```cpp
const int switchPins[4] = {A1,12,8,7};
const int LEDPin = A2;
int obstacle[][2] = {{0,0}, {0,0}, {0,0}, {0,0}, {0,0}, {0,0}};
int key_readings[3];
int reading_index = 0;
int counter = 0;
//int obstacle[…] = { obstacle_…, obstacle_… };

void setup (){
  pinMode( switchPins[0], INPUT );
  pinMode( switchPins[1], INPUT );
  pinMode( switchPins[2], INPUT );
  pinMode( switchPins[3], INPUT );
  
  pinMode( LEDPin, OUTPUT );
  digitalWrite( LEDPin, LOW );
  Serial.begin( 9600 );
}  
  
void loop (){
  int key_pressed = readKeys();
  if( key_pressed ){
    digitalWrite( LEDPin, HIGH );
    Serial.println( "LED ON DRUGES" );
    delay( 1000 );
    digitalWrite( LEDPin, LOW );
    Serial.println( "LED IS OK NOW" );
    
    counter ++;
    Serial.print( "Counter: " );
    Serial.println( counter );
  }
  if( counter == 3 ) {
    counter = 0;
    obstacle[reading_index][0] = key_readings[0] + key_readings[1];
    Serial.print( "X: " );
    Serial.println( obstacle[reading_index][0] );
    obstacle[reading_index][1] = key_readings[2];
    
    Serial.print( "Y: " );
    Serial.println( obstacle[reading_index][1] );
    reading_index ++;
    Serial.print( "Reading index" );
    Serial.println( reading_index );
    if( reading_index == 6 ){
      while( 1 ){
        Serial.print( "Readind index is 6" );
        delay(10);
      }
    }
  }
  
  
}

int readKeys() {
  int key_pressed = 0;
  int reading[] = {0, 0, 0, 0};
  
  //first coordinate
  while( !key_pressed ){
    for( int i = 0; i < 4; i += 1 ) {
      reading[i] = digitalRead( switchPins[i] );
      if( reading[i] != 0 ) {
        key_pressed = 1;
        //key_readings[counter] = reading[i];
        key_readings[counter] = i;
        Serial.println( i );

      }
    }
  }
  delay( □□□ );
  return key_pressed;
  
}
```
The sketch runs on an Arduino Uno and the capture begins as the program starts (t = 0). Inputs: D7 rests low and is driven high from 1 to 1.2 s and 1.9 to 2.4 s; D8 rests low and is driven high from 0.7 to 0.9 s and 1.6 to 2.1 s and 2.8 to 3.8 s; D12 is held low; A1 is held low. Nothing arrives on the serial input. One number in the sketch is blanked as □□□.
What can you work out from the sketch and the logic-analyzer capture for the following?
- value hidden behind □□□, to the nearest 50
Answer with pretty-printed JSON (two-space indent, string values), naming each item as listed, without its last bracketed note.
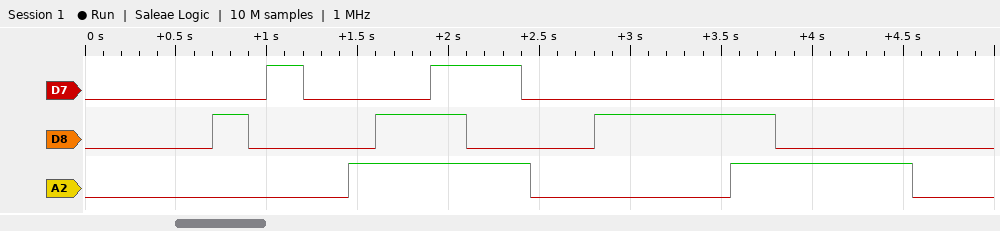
{
  "value hidden behind □□□, to the nearest 50": "750"
}
